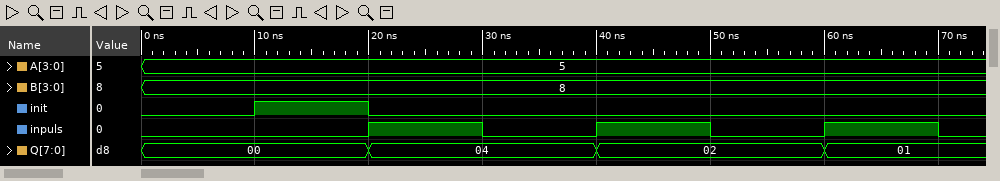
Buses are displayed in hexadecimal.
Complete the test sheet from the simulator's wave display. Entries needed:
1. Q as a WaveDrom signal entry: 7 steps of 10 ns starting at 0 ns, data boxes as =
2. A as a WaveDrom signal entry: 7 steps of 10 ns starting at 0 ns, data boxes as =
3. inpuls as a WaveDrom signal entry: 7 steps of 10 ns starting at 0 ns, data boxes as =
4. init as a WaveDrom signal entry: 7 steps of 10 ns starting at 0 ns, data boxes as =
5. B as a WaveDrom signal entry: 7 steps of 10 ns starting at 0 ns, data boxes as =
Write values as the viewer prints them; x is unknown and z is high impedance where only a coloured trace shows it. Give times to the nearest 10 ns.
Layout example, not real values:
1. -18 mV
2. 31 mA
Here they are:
1. {name: 'Q', wave: '=.=.=.=', data: '00 04 02 01'}
2. {name: 'A', wave: '=......', data: '5'}
3. {name: 'inpuls', wave: '0.10101'}
4. {name: 'init', wave: '010....'}
5. {name: 'B', wave: '=......', data: '8'}
